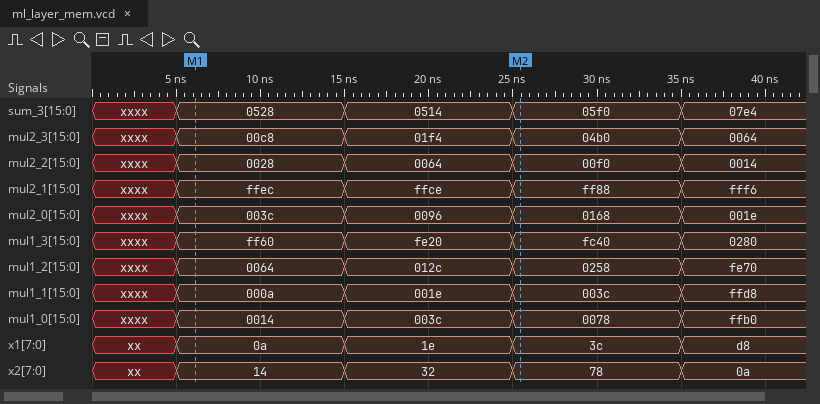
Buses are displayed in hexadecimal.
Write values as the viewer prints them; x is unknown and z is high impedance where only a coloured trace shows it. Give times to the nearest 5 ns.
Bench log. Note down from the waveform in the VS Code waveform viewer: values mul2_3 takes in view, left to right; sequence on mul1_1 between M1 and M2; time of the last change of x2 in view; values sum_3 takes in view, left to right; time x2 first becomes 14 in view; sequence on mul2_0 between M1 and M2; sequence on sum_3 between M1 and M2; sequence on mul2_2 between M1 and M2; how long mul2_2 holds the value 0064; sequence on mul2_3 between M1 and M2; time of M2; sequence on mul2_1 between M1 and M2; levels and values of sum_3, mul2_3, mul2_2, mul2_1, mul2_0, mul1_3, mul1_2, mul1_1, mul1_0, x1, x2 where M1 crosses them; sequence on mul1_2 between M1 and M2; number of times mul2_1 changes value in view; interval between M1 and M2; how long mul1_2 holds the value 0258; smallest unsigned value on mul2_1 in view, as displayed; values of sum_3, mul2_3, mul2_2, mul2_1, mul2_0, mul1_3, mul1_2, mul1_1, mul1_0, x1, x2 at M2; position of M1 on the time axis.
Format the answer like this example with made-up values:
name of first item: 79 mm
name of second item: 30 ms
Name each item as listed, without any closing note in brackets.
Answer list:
values mul2_3 takes in view, left to right: xxxx, 00c8, 01f4, 04b0, 0064
sequence on mul1_1 between M1 and M2: 000a, 001e, 003c
time of the last change of x2 in view: 35 ns
values sum_3 takes in view, left to right: xxxx, 0528, 0514, 05f0, 07e4
time x2 first becomes 14 in view: 5 ns
sequence on mul2_0 between M1 and M2: 003c, 0096, 0168
sequence on sum_3 between M1 and M2: 0528, 0514, 05f0
sequence on mul2_2 between M1 and M2: 0028, 0064, 00f0
how long mul2_2 holds the value 0064: 10 ns
sequence on mul2_3 between M1 and M2: 00c8, 01f4, 04b0
time of M2: 25 ns
sequence on mul2_1 between M1 and M2: ffec, ffce, ff88
levels and values of sum_3, mul2_3, mul2_2, mul2_1, mul2_0, mul1_3, mul1_2, mul1_1, mul1_0, x1, x2 where M1 crosses them: sum_3=0528, mul2_3=00c8, mul2_2=0028, mul2_1=ffec, mul2_0=003c, mul1_3=ff60, mul1_2=0064, mul1_1=000a, mul1_0=0014, x1=0a, x2=14
sequence on mul1_2 between M1 and M2: 0064, 012c, 0258
number of times mul2_1 changes value in view: 4
interval between M1 and M2: 20 ns
how long mul1_2 holds the value 0258: 10 ns
smallest unsigned value on mul2_1 in view, as displayed: ff88
values of sum_3, mul2_3, mul2_2, mul2_1, mul2_0, mul1_3, mul1_2, mul1_1, mul1_0, x1, x2 at M2: sum_3=05f0, mul2_3=04b0, mul2_2=00f0, mul2_1=ff88, mul2_0=0168, mul1_3=fc40, mul1_2=0258, mul1_1=003c, mul1_0=0078, x1=3c, x2=78
position of M1 on the time axis: 5 ns
